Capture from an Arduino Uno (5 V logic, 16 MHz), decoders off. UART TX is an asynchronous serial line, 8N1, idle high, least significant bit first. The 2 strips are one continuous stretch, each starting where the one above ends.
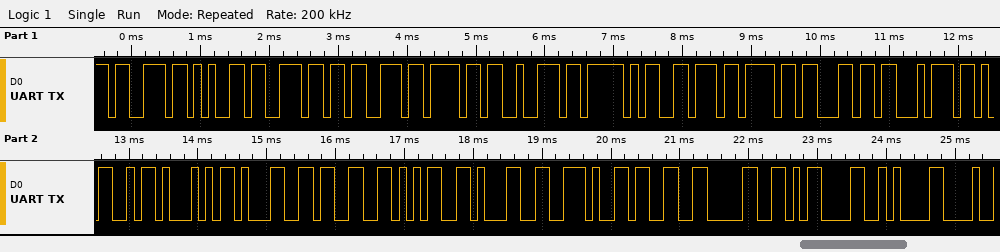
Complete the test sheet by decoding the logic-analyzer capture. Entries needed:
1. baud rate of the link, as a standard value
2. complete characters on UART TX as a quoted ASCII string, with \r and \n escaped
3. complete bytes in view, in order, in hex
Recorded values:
9600 baud
"sensor_voltMQ1351.30\r\n"
73 65 6E 73 6F 72 5F 76 6F 6C 74 4D 51 31 33 35 31 2E 33 30 0D 0A
